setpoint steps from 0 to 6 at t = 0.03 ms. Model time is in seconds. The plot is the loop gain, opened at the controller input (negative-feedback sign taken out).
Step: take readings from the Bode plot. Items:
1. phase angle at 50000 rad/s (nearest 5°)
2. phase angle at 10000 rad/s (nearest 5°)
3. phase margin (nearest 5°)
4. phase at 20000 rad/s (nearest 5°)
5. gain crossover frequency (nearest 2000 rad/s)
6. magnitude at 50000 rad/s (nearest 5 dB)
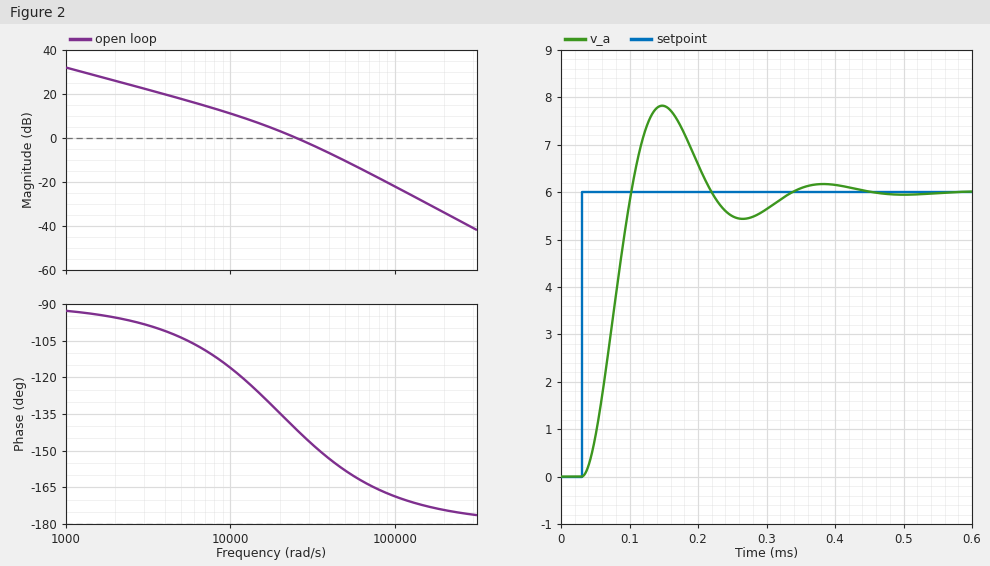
-160°
-115°
40°
-135°
26000 rad/s
-10 dB
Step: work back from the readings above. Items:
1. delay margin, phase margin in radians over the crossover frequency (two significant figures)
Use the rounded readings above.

0.000027 s
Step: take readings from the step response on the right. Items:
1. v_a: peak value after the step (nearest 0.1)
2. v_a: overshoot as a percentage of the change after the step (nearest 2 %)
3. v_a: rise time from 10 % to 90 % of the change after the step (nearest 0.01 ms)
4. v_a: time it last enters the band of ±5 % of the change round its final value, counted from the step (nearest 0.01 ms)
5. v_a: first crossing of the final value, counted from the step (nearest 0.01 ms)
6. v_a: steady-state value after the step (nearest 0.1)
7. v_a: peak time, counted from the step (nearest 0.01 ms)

7.8
30 %
0.05 ms
0.28 ms
0.07 ms
6.0
0.12 ms
